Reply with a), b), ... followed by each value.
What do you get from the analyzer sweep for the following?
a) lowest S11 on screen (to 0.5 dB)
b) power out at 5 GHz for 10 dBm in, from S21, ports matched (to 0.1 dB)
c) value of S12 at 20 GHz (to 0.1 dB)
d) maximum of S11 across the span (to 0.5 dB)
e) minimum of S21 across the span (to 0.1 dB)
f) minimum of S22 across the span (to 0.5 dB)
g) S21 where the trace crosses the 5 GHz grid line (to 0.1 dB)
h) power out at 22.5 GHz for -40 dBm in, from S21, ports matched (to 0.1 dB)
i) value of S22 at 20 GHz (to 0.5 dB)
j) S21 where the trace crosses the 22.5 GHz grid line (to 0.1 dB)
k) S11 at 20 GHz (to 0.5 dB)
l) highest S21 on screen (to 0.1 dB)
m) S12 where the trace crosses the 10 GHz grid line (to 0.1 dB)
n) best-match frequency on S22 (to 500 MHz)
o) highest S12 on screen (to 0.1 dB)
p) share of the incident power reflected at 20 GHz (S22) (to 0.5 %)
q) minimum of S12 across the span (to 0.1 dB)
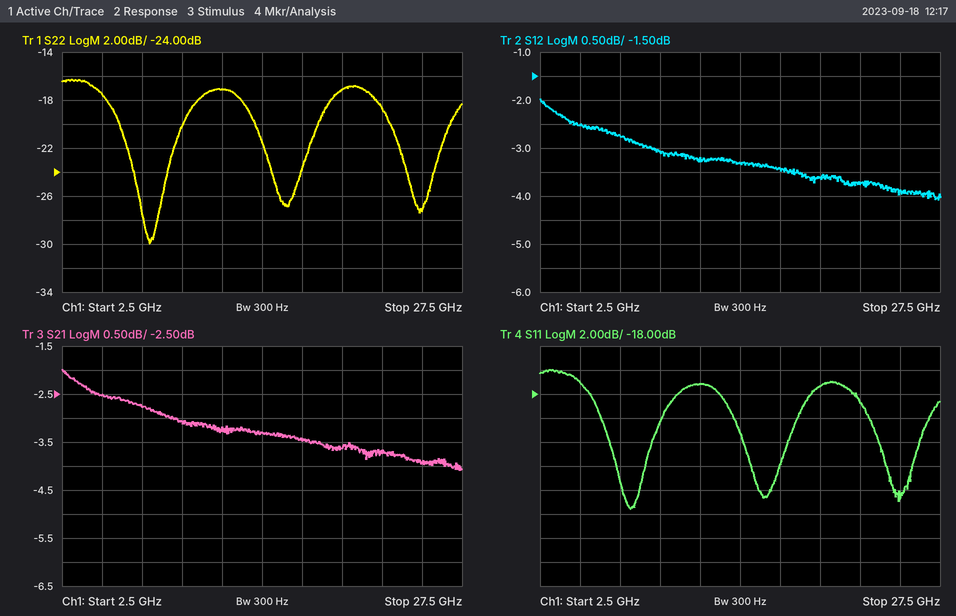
a) -27.5 dB
b) 7.5 dBm
c) -3.6 dB
d) -16.0 dB
e) -4.1 dB
f) -30.0 dB
g) -2.5 dB
h) -43.7 dBm
i) -17.0 dB
j) -3.7 dB
k) -17.5 dB
l) -2.0 dB
m) -3.1 dB
n) 8.0 GHz
o) -2.0 dB
p) 2.0 %
q) -4.1 dB
